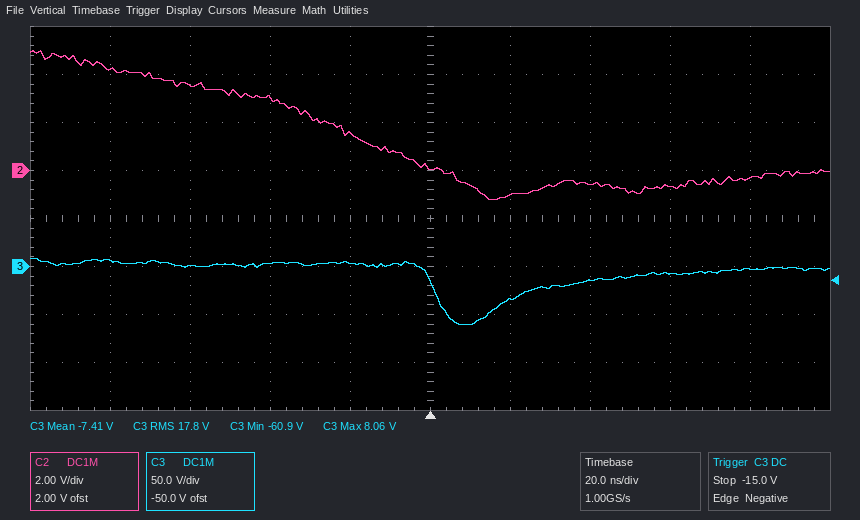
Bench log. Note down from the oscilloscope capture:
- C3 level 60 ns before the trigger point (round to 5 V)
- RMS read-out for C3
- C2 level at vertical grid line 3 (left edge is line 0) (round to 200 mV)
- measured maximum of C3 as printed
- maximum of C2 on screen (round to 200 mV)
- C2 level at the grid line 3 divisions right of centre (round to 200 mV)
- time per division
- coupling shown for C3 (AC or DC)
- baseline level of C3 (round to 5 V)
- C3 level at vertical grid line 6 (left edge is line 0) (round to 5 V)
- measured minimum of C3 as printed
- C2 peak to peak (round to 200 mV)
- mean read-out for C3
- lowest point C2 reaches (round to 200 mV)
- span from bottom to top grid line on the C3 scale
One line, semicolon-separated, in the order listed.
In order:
0 V; 17.8 V; 3.0 V; 8.06 V; 5.0 V; -600 mV; 20 ns; DC; 0 V; -35 V; -60.9 V; 6.2 V; -7.41 V; -1.2 V; 400 V
